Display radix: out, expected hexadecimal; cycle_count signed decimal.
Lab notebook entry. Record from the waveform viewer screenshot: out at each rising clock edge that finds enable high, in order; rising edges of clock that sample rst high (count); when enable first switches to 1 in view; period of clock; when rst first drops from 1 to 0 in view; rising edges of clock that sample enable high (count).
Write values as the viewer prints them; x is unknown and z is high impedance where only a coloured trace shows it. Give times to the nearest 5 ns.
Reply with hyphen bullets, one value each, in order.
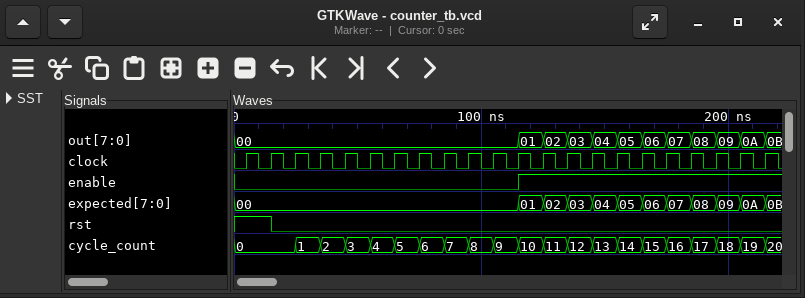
- 01, 02, 03, 04, 05, 06, 07, 08, 09, 0A
- 2
- 115 ns
- 10 ns
- 15 ns
- 10
